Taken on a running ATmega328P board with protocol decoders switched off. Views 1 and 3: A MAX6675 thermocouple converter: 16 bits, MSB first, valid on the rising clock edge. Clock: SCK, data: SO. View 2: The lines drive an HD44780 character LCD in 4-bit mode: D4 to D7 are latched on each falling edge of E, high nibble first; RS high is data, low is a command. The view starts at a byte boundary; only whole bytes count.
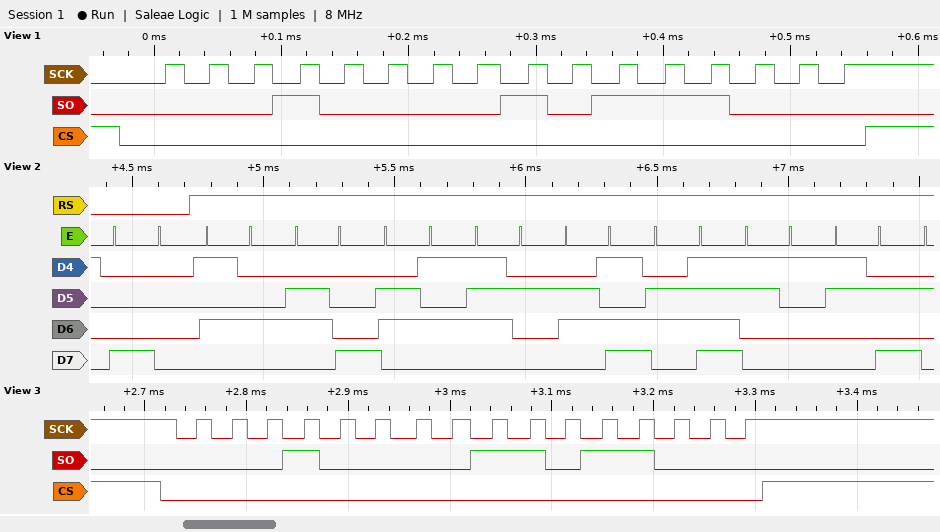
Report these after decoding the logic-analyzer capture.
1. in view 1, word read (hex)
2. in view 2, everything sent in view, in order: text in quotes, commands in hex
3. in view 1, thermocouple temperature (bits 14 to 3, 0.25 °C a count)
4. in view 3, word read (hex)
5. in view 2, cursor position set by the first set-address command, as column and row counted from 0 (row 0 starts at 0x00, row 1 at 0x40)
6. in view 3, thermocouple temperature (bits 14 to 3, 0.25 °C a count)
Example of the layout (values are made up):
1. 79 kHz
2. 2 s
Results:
1. 0x10B8
2. 0x80 "Thermo1:"
3. 133.75 °C
4. 0x10D8
5. column 0, row 0
6. 134.75 °C
